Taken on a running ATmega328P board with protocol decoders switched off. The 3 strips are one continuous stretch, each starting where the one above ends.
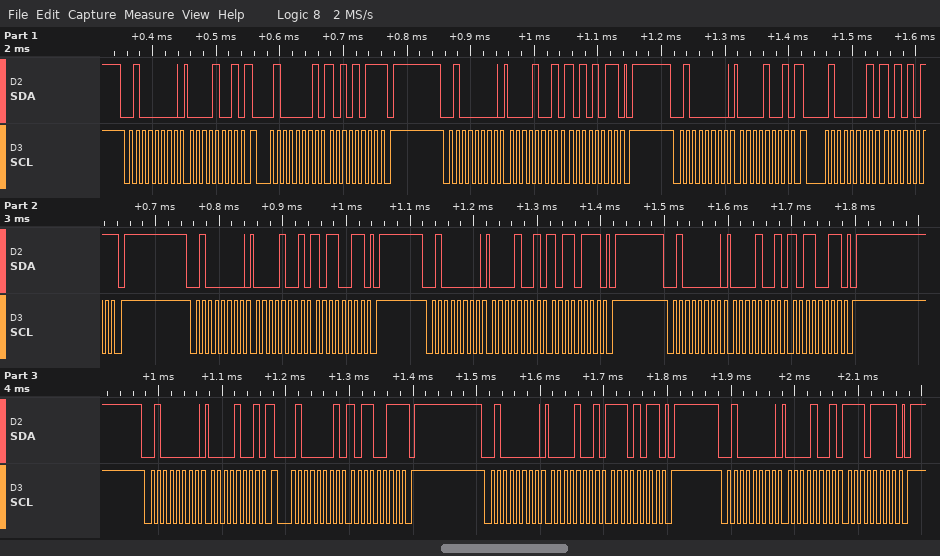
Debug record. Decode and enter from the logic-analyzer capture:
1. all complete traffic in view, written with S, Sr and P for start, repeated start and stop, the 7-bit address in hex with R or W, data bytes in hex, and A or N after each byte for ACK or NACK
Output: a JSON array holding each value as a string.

["S 20W A 09 A Sr 20R A AB N P S 20W A 09 A AB A P S 20W A 09 A Sr 20R A AB N P S 20W A 09 A B3 A P S 20W A 09 A B7 A P S 20W A 09 A B3 A P S 20W A 09 A Sr 20R A B3 N P S 20W A 09 A EB A P S 20W A 09 A EF A P"]
